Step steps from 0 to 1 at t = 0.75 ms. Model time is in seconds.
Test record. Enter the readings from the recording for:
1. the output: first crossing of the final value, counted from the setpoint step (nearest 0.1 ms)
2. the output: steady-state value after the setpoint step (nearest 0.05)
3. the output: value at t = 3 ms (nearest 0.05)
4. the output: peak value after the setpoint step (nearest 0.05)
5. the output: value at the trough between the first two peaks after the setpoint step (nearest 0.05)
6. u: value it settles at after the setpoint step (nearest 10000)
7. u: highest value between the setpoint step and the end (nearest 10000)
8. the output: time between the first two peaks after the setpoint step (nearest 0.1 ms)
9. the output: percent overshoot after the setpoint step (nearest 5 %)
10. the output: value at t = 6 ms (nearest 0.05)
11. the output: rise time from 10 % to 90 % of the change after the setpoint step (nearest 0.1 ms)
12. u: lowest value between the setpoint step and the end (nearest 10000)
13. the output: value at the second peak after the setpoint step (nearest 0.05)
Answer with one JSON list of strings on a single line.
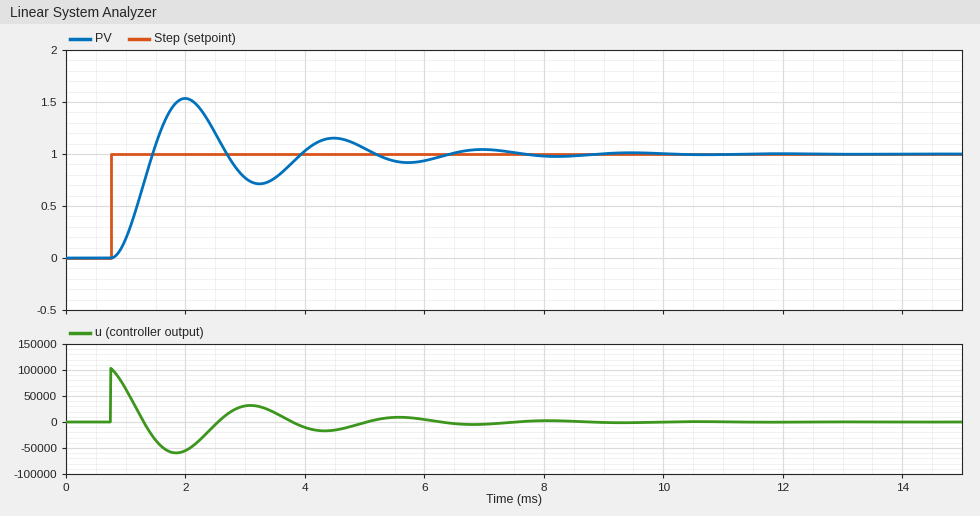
["0.7 ms", "1.00", "0.75", "1.55", "0.70", "0", "100000", "2.5 ms", "55 %", "0.95", "0.5 ms", "-60000", "1.15"]
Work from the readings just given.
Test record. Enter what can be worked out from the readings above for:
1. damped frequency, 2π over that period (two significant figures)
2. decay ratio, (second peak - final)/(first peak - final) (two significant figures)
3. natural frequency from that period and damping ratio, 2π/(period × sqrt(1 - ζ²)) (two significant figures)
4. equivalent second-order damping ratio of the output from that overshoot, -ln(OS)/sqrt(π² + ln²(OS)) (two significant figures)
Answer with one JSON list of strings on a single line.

["2.5 rad/ms", "0.27", "2.6 rad/ms", "0.19"]
